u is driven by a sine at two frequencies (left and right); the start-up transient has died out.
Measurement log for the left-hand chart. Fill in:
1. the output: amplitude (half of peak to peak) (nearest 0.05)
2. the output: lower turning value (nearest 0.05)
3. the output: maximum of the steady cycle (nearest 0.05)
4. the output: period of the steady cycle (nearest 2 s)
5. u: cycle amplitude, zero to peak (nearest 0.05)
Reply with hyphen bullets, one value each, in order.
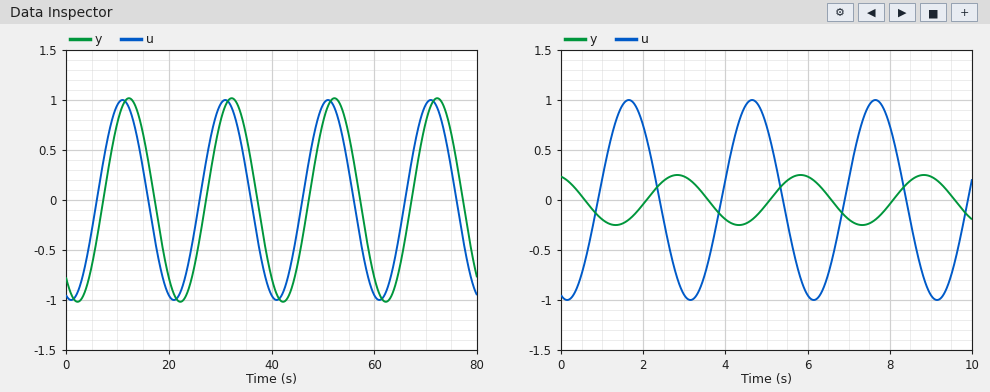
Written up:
- 1.00
- -1.00
- 1.00
- 20 s
- 1.00
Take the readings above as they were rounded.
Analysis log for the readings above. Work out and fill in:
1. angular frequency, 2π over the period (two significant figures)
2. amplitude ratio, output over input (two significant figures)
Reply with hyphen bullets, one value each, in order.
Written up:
- 0.31 rad/s
- 1.0
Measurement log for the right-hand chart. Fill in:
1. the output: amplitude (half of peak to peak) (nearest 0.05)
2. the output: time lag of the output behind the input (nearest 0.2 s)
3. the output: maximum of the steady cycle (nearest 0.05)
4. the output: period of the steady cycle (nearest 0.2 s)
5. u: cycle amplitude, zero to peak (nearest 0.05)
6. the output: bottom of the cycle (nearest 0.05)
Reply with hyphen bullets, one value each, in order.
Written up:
- 0.25
- 1.2 s
- 0.25
- 3.0 s
- 1.00
- -0.25
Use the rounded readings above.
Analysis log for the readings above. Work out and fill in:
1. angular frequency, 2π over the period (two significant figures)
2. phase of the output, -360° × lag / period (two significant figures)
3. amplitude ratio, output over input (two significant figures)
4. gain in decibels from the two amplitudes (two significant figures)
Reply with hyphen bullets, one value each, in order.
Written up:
- 2.1 rad/s
- -140°
- 0.25
- -12 dB
